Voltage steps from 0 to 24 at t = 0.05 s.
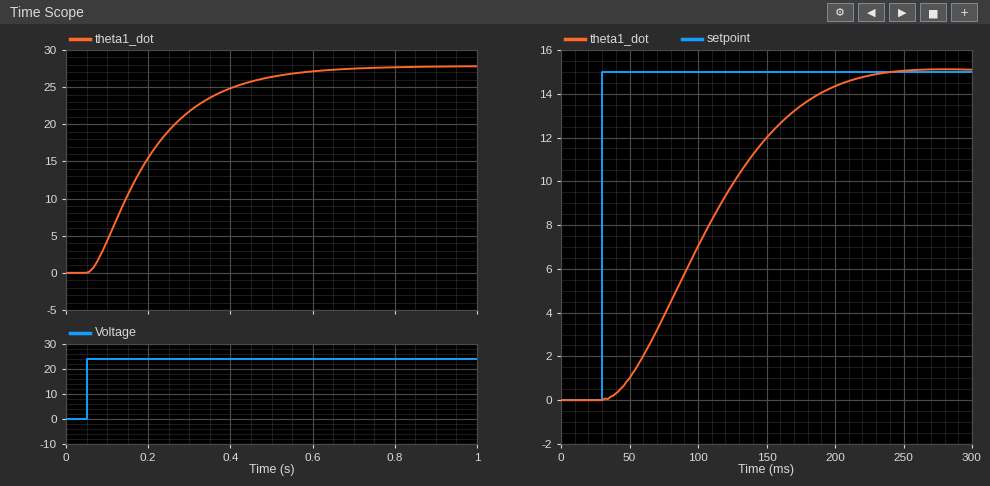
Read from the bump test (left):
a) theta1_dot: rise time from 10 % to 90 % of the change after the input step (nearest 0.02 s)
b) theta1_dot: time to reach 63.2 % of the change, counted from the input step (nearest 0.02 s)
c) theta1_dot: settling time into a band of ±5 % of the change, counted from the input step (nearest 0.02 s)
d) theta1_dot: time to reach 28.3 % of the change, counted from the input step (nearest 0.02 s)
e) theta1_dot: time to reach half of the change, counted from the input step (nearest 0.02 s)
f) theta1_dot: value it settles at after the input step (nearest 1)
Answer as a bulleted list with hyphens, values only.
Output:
- 0.32 s
- 0.18 s
- 0.46 s
- 0.08 s
- 0.14 s
- 28
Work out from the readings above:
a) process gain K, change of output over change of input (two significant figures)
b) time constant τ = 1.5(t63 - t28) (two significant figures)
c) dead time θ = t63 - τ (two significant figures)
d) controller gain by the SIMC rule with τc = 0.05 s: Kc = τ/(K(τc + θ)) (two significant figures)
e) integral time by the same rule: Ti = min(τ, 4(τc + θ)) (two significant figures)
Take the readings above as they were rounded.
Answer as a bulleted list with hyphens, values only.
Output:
- 1.2
- 0.15 s
- 0.030 s
- 1.6
- 0.15 s
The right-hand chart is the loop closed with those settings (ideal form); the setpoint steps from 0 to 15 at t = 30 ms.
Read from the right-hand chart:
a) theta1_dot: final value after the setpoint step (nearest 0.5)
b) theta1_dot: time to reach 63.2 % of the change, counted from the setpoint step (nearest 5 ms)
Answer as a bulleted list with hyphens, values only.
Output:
- 15.0
- 90 ms
